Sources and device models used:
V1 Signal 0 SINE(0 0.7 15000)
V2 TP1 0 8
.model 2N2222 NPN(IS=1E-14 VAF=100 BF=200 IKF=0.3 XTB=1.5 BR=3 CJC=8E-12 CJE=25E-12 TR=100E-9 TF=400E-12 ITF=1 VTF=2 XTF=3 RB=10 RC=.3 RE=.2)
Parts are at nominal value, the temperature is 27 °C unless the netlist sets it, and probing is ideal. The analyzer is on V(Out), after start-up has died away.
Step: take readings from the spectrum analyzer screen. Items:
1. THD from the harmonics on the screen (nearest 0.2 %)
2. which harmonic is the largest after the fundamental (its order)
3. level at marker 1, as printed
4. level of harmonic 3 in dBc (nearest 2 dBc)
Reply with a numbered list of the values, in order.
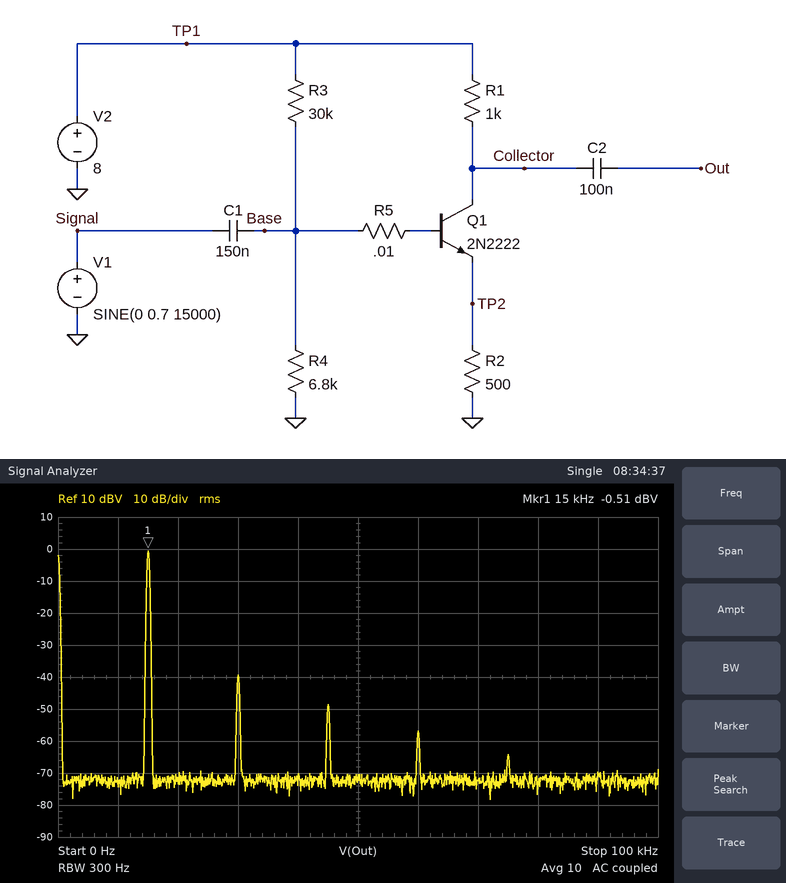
1. 1.2 %
2. 2
3. -0.51 dBV
4. -48 dBc
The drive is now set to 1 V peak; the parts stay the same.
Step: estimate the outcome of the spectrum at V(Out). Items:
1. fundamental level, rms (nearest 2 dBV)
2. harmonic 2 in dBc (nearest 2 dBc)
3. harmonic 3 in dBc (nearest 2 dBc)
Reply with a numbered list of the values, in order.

1. 2 dBV
2. -26 dBc
3. -30 dBc
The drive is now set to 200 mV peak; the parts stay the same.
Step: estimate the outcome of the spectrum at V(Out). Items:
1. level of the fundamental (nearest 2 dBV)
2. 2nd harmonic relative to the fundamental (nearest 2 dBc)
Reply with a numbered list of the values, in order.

1. -12 dBV
2. -54 dBc
